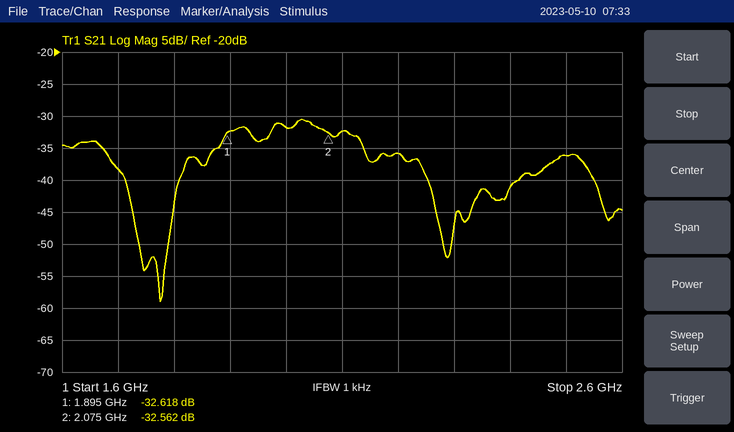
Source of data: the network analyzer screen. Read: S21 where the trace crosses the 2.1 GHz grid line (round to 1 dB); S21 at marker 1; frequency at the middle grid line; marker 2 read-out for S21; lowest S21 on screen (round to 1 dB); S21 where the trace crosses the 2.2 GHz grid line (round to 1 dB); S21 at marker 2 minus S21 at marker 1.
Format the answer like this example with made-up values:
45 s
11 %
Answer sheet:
-32 dB
-32.618 dB
2.1 GHz
-32.562 dB
-59 dB
-36 dB
0.056 dB
